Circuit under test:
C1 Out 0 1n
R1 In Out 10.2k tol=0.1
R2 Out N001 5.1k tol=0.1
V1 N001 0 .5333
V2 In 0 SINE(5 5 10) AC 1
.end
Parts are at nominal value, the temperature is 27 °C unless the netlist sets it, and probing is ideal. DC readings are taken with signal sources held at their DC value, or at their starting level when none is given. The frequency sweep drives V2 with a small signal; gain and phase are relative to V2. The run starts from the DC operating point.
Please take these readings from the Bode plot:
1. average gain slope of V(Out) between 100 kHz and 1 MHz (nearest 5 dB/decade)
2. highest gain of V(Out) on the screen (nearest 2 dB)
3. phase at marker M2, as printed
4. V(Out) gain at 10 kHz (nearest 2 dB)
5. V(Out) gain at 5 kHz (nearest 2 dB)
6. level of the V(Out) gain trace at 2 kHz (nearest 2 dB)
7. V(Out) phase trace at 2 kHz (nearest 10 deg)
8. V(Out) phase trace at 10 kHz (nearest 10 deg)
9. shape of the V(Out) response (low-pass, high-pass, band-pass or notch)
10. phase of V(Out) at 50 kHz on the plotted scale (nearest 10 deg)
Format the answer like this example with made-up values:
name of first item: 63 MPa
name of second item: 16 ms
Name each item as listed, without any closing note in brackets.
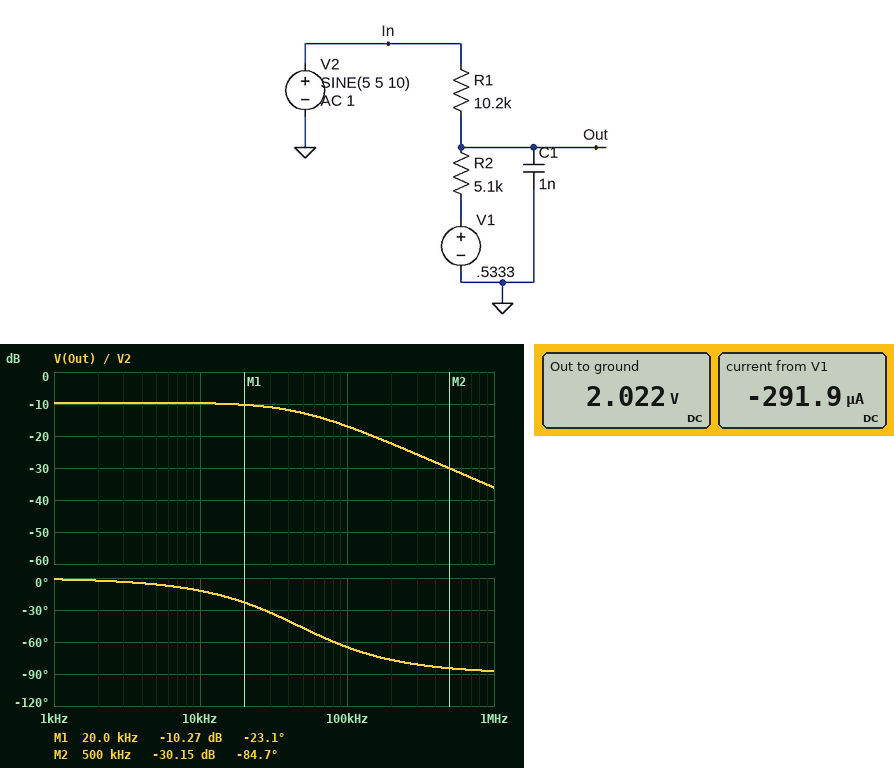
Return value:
average gain slope of V(Out) between 100 kHz and 1 MHz: -20 dB/decade
highest gain of V(Out) on the screen: -10 dB
phase at marker M2, as printed: -84.7 deg
V(Out) gain at 10 kHz: -10 dB
V(Out) gain at 5 kHz: -10 dB
level of the V(Out) gain trace at 2 kHz: -10 dB
V(Out) phase trace at 2 kHz: 0 deg
V(Out) phase trace at 10 kHz: -10 deg
shape of the V(Out) response: low-pass
phase of V(Out) at 50 kHz on the plotted scale: -50 deg
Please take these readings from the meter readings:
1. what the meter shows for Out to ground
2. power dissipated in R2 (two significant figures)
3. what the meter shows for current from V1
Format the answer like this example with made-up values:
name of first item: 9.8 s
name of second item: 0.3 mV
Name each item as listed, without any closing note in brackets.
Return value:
what the meter shows for Out to ground: 2.022 V
power dissipated in R2: 430 µW
what the meter shows for current from V1: -291.9 µA
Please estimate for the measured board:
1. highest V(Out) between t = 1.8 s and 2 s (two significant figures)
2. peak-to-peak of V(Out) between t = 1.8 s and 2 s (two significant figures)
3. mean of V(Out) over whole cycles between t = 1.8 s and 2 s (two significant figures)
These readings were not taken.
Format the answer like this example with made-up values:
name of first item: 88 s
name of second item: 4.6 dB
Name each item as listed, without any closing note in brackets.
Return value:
highest V(Out) between t = 1.8 s and 2 s: 3.7 V
peak-to-peak of V(Out) between t = 1.8 s and 2 s: 3.3 V
mean of V(Out) over whole cycles between t = 1.8 s and 2 s: 2.0 V
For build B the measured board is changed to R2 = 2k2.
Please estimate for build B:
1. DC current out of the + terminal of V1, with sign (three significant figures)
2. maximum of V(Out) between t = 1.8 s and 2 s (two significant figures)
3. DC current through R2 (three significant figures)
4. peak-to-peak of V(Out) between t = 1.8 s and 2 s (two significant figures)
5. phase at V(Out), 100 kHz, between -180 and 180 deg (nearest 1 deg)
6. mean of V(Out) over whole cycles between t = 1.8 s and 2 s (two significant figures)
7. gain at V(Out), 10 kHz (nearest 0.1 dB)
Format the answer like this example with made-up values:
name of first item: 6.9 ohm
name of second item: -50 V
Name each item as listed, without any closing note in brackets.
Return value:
DC current out of the + terminal of V1, with sign: -360 µA
maximum of V(Out) between t = 1.8 s and 2 s: 2.2 V
DC current through R2: 360 µA
peak-to-peak of V(Out) between t = 1.8 s and 2 s: 1.8 V
phase at V(Out), 100 kHz, between -180 and 180 deg: -49 deg
mean of V(Out) over whole cycles between t = 1.8 s and 2 s: 1.3 V
gain at V(Out), 10 kHz: -15.1 dB
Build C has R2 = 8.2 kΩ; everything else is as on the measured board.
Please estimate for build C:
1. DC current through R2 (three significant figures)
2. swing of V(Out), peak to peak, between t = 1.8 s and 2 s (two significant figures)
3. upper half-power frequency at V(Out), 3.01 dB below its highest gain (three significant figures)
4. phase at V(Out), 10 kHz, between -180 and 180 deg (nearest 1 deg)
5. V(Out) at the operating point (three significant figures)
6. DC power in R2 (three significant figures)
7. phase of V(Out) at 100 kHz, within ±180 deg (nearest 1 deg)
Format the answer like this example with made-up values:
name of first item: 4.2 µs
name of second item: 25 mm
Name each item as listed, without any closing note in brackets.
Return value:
DC current through R2: 243 µA
swing of V(Out), peak to peak, between t = 1.8 s and 2 s: 4.5 V
upper half-power frequency at V(Out), 3.01 dB below its highest gain: 35.0 kHz
phase at V(Out), 10 kHz, between -180 and 180 deg: -16 deg
V(Out) at the operating point: 2.52 V
DC power in R2: 483 µW
phase of V(Out) at 100 kHz, within ±180 deg: -71 deg
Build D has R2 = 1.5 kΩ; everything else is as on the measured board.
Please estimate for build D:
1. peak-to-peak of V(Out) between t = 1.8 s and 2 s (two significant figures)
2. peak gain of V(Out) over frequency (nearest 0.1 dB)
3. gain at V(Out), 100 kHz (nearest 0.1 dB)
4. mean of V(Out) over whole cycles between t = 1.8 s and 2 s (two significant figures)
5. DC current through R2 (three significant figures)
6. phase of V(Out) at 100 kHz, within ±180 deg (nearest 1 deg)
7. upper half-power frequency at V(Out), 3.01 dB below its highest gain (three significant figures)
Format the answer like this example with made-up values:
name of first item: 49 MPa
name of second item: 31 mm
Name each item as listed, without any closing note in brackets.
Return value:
peak-to-peak of V(Out) between t = 1.8 s and 2 s: 1.3 V
peak gain of V(Out) over frequency: -17.8 dB
gain at V(Out), 100 kHz: -20.1 dB
mean of V(Out) over whole cycles between t = 1.8 s and 2 s: 1.1 V
DC current through R2: 382 µA
phase of V(Out) at 100 kHz, within ±180 deg: -39 deg
upper half-power frequency at V(Out), 3.01 dB below its highest gain: 122 kHz
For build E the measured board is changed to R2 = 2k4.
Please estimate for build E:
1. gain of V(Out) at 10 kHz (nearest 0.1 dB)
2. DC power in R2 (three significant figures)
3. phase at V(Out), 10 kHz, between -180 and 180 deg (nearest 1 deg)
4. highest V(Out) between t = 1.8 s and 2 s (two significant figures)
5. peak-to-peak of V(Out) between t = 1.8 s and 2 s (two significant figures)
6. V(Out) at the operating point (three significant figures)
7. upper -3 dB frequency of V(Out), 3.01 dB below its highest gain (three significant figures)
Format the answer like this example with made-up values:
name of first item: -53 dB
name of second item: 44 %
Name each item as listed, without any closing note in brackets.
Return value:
gain of V(Out) at 10 kHz: -14.5 dB
DC power in R2: 302 µW
phase at V(Out), 10 kHz, between -180 and 180 deg: -7 deg
highest V(Out) between t = 1.8 s and 2 s: 2.3 V
peak-to-peak of V(Out) between t = 1.8 s and 2 s: 1.9 V
V(Out) at the operating point: 1.38 V
upper -3 dB frequency of V(Out), 3.01 dB below its highest gain: 81.9 kHz
